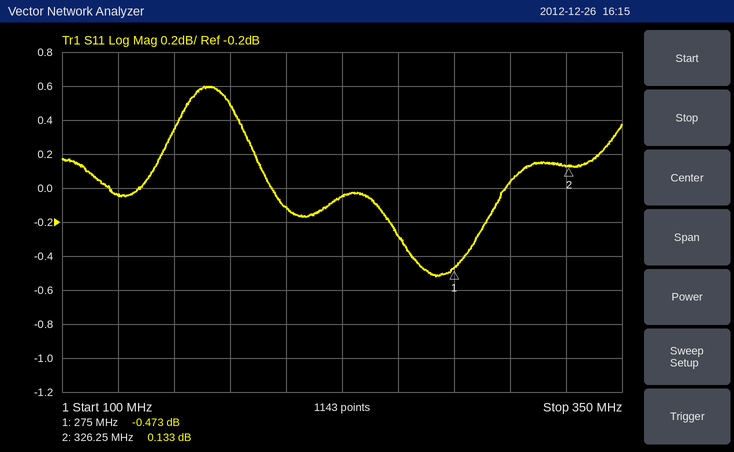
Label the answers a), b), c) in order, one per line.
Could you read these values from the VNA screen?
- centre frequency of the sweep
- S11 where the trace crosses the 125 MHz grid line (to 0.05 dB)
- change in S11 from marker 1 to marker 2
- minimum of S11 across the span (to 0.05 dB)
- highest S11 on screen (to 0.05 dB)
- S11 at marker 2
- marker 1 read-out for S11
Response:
a) 225 MHz
b) -0.05 dB
c) 0.606 dB
d) -0.50 dB
e) 0.60 dB
f) 0.133 dB
g) -0.473 dB
